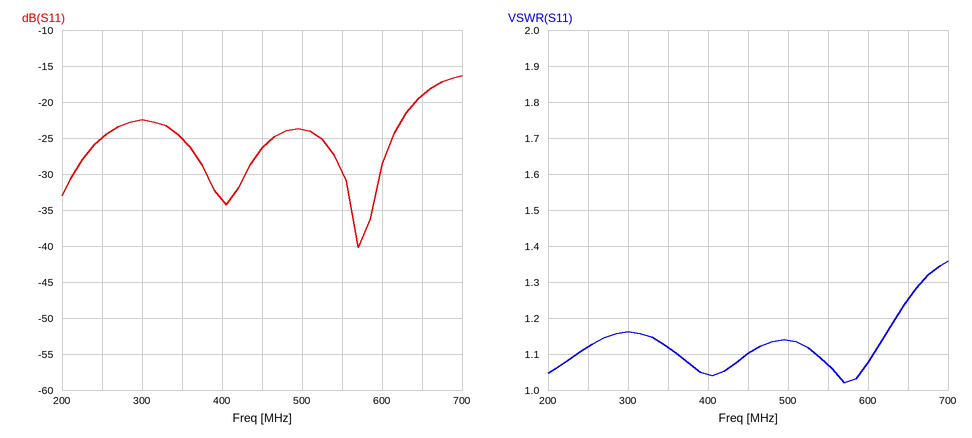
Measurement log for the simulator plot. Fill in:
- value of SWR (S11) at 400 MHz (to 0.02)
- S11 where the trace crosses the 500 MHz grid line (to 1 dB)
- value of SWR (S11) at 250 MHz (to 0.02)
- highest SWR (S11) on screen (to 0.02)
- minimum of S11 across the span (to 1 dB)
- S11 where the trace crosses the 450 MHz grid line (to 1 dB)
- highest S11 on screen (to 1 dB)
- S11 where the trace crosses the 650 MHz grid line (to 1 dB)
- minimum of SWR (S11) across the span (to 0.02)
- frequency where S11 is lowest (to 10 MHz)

1.04
-24 dB
1.12
1.36
-40 dB
-26 dB
-16 dB
-19 dB
1.02
570 MHz
